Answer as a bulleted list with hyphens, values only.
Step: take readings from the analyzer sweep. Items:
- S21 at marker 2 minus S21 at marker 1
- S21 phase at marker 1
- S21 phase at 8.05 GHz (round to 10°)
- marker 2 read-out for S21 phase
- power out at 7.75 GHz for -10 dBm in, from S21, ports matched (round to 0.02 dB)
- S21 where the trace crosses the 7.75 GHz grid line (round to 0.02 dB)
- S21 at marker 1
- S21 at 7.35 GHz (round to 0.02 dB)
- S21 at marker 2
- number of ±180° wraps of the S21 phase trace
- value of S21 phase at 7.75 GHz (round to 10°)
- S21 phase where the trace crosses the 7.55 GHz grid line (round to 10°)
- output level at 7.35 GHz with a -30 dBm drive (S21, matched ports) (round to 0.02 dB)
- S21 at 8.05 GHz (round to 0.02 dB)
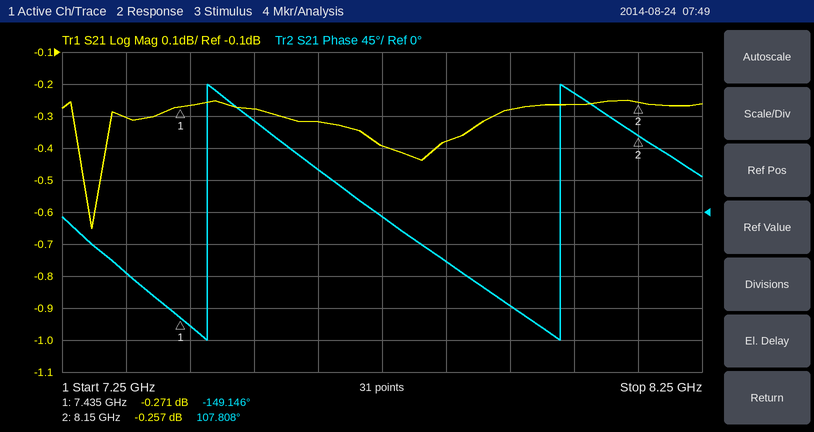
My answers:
- 0.014 dB
- -149.146°
- 170°
- 107.808°
- -10.40 dBm
- -0.40 dB
- -0.271 dB
- -0.30 dB
- -0.257 dB
- 2
- -10°
- 130°
- -30.30 dBm
- -0.26 dB
